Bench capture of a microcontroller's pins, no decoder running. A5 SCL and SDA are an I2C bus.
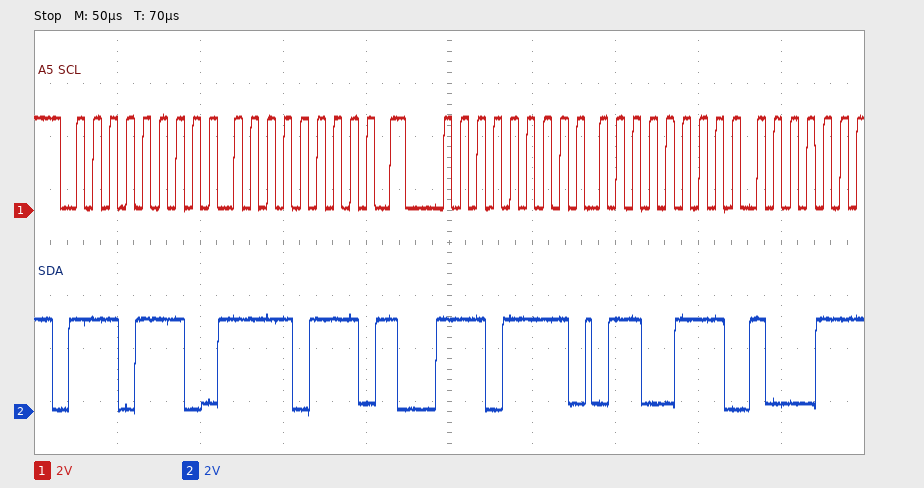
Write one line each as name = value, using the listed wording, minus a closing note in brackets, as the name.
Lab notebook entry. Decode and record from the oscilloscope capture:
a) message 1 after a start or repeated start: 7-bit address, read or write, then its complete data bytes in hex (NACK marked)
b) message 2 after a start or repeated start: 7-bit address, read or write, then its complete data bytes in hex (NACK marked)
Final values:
message 1 after a start or repeated start: 7-bit address, read or write, then its complete data bytes in hex = 0x77 write: F7
message 2 after a start or repeated start: 7-bit address, read or write, then its complete data bytes in hex = 0x77 read: 67
